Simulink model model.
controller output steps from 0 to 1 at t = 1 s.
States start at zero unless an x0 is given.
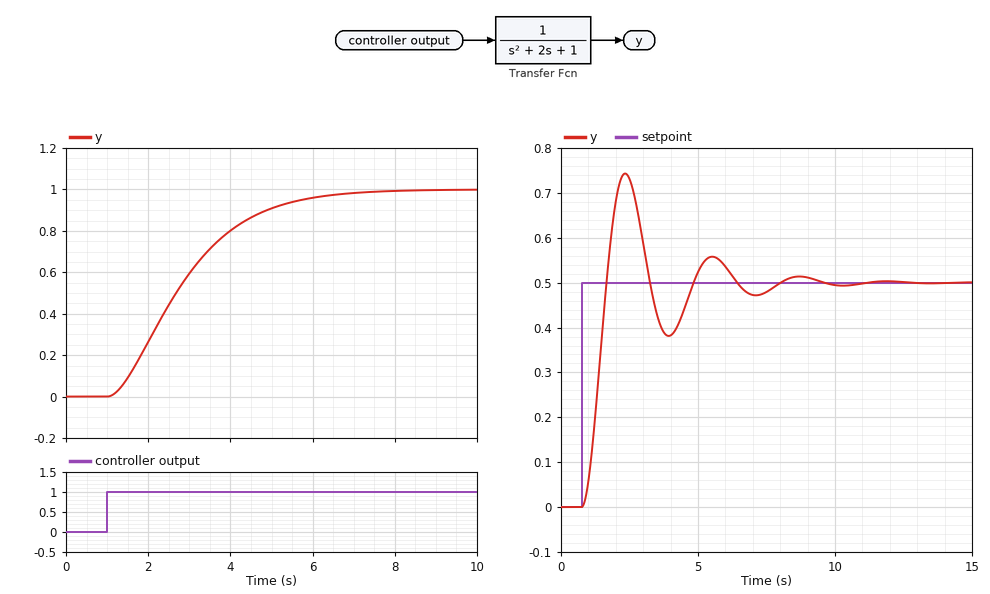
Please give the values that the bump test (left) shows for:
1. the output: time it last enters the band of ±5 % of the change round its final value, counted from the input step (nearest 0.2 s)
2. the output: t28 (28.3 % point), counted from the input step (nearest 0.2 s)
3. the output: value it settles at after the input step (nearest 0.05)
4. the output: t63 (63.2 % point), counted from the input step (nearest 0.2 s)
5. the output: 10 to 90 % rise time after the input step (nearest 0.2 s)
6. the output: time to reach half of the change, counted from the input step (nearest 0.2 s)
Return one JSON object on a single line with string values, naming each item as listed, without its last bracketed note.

{"the output: time it last enters the band of ±5 % of the change round its final value, counted from the input step": "4.8 s", "the output: t28 (28.3 % point), counted from the input step": "1.0 s", "the output: value it settles at after the input step": "1.00", "the output: t63 (63.2 % point), counted from the input step": "2.2 s", "the output: 10 to 90 % rise time after the input step": "3.4 s", "the output: time to reach half of the change, counted from the input step": "1.6 s"}
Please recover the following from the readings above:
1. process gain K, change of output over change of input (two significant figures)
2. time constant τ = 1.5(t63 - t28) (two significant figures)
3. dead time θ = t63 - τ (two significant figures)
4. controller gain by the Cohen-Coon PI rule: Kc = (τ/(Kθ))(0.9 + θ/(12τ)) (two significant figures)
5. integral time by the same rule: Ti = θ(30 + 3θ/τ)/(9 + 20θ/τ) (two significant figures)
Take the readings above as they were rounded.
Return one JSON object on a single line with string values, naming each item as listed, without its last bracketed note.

{"process gain K, change of output over change of input": "1.0", "time constant τ = 1.5(t63 - t28)": "1.8 s", "dead time θ = t63 - τ": "0.40 s", "controller gain by the Cohen-Coon PI rule: Kc = (τ/(Kθ))(0.9 + θ/(12τ))": "4.1", "integral time by the same rule: Ti = θ(30 + 3θ/τ)/(9 + 20θ/τ)": "0.91 s"}
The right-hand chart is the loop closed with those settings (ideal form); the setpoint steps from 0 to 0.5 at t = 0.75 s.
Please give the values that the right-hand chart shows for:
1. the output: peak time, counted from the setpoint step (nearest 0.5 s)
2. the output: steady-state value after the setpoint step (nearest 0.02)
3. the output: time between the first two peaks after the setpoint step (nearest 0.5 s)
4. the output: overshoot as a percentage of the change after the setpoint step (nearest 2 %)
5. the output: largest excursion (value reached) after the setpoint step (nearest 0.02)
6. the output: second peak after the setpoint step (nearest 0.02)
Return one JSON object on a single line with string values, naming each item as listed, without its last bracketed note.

{"the output: peak time, counted from the setpoint step": "1.5 s", "the output: steady-state value after the setpoint step": "0.50", "the output: time between the first two peaks after the setpoint step": "3.0 s", "the output: overshoot as a percentage of the change after the setpoint step": "48 %", "the output: largest excursion (value reached) after the setpoint step": "0.74", "the output: second peak after the setpoint step": "0.56"}
